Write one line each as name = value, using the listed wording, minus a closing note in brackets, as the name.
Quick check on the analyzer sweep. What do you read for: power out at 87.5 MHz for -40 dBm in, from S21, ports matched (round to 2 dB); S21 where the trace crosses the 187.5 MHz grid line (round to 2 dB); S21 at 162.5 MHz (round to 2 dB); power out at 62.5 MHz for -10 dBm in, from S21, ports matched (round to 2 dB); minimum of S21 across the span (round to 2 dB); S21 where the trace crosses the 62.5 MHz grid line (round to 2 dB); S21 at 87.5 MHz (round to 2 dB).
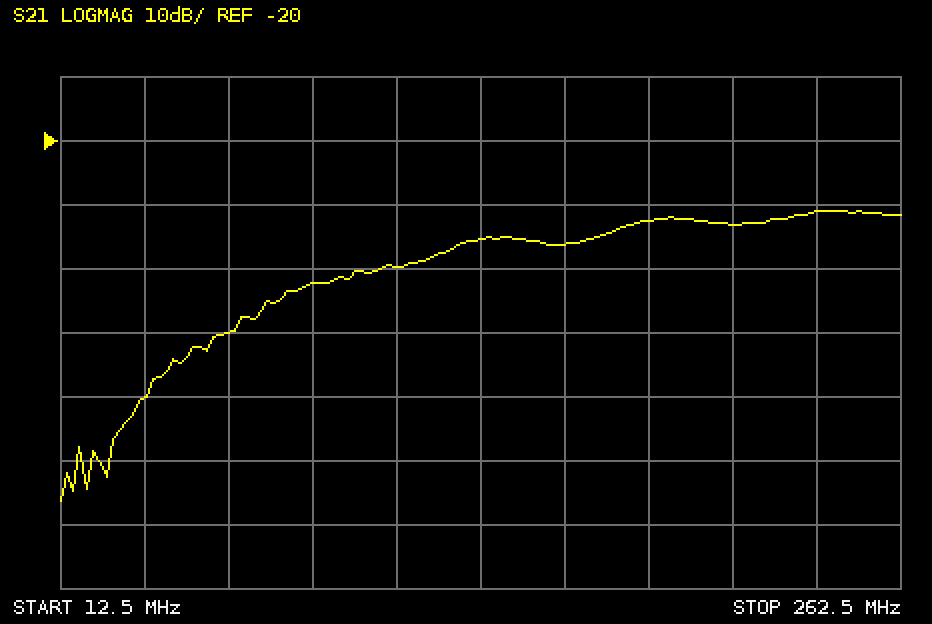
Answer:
power out at 87.5 MHz for -40 dBm in, from S21, ports matched = -82 dBm
S21 where the trace crosses the 187.5 MHz grid line = -32 dB
S21 at 162.5 MHz = -36 dB
power out at 62.5 MHz for -10 dBm in, from S21, ports matched = -60 dBm
minimum of S21 across the span = -76 dB
S21 where the trace crosses the 62.5 MHz grid line = -50 dB
S21 at 87.5 MHz = -42 dB
